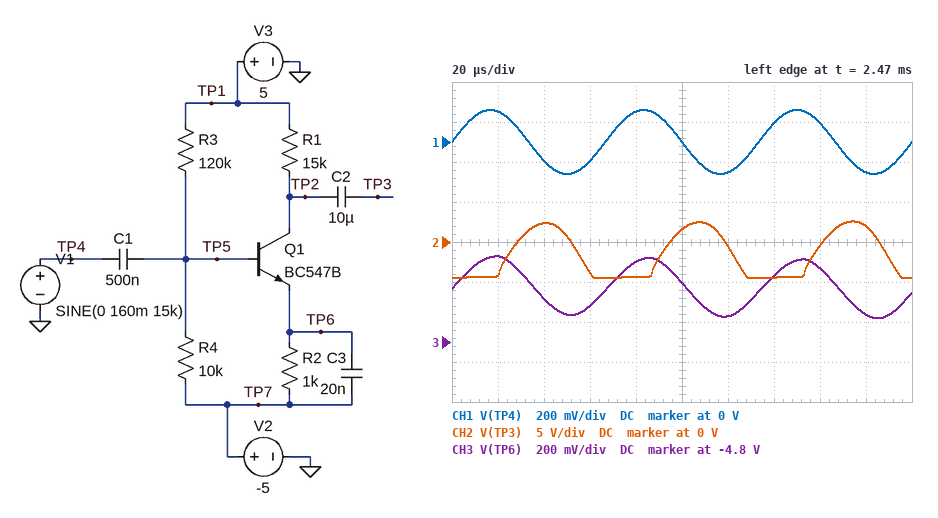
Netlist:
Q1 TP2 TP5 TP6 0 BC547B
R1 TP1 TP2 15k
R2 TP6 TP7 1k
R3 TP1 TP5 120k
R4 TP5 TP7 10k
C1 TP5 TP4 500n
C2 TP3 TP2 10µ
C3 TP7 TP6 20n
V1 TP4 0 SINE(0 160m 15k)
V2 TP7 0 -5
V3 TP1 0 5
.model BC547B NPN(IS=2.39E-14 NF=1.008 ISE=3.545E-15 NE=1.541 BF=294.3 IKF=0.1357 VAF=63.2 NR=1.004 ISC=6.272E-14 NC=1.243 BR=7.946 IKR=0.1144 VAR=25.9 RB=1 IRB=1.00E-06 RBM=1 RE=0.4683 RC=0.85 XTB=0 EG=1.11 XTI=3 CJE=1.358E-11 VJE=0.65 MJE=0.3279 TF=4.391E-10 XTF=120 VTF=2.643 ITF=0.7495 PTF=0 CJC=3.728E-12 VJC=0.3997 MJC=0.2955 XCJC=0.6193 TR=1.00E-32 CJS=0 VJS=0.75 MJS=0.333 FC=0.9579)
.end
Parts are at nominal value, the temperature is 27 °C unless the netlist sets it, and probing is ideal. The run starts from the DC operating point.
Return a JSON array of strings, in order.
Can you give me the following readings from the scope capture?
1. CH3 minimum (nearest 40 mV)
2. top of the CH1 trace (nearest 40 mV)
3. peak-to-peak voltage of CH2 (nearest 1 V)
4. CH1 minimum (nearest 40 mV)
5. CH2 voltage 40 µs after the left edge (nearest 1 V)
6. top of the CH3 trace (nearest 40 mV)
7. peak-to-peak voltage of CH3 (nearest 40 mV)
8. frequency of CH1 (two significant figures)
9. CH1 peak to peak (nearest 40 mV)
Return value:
["-4.68 V", "160 mV", "7 V", "-160 mV", "2 V", "-4.36 V", "320 mV", "15 kHz", "320 mV"]
